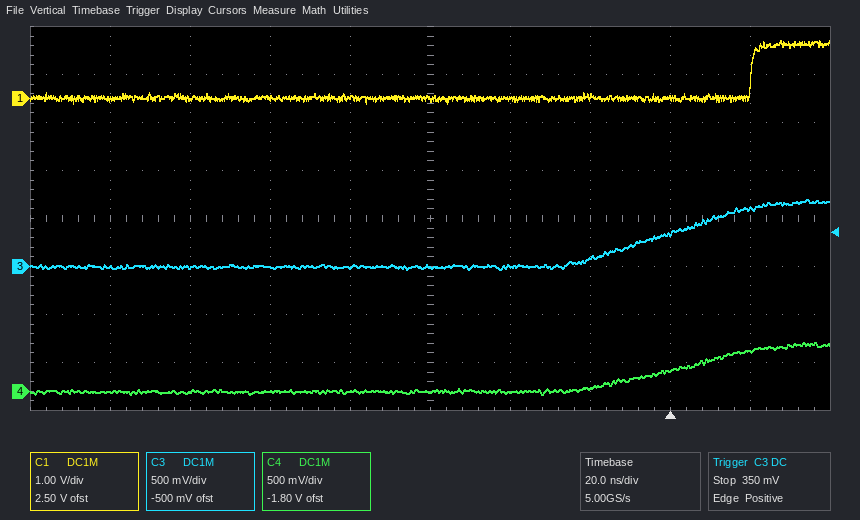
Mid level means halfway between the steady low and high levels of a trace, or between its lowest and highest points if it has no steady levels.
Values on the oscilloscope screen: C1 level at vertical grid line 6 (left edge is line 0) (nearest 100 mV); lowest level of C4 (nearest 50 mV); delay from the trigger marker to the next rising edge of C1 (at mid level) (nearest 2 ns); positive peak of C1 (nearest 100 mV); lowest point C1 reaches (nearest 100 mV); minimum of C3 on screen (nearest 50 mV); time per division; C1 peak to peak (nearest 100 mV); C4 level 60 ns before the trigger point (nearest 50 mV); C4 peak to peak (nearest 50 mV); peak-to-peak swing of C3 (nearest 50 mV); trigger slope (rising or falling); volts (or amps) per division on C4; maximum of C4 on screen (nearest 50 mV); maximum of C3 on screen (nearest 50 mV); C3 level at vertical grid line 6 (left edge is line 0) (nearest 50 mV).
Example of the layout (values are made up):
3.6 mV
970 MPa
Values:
0.0 V
-50 mV
20 ns
1.2 V
-100 mV
-50 mV
20 ns
1.3 V
0 mV
550 mV
750 mV
rising
500 mV
500 mV
700 mV
0 mV
